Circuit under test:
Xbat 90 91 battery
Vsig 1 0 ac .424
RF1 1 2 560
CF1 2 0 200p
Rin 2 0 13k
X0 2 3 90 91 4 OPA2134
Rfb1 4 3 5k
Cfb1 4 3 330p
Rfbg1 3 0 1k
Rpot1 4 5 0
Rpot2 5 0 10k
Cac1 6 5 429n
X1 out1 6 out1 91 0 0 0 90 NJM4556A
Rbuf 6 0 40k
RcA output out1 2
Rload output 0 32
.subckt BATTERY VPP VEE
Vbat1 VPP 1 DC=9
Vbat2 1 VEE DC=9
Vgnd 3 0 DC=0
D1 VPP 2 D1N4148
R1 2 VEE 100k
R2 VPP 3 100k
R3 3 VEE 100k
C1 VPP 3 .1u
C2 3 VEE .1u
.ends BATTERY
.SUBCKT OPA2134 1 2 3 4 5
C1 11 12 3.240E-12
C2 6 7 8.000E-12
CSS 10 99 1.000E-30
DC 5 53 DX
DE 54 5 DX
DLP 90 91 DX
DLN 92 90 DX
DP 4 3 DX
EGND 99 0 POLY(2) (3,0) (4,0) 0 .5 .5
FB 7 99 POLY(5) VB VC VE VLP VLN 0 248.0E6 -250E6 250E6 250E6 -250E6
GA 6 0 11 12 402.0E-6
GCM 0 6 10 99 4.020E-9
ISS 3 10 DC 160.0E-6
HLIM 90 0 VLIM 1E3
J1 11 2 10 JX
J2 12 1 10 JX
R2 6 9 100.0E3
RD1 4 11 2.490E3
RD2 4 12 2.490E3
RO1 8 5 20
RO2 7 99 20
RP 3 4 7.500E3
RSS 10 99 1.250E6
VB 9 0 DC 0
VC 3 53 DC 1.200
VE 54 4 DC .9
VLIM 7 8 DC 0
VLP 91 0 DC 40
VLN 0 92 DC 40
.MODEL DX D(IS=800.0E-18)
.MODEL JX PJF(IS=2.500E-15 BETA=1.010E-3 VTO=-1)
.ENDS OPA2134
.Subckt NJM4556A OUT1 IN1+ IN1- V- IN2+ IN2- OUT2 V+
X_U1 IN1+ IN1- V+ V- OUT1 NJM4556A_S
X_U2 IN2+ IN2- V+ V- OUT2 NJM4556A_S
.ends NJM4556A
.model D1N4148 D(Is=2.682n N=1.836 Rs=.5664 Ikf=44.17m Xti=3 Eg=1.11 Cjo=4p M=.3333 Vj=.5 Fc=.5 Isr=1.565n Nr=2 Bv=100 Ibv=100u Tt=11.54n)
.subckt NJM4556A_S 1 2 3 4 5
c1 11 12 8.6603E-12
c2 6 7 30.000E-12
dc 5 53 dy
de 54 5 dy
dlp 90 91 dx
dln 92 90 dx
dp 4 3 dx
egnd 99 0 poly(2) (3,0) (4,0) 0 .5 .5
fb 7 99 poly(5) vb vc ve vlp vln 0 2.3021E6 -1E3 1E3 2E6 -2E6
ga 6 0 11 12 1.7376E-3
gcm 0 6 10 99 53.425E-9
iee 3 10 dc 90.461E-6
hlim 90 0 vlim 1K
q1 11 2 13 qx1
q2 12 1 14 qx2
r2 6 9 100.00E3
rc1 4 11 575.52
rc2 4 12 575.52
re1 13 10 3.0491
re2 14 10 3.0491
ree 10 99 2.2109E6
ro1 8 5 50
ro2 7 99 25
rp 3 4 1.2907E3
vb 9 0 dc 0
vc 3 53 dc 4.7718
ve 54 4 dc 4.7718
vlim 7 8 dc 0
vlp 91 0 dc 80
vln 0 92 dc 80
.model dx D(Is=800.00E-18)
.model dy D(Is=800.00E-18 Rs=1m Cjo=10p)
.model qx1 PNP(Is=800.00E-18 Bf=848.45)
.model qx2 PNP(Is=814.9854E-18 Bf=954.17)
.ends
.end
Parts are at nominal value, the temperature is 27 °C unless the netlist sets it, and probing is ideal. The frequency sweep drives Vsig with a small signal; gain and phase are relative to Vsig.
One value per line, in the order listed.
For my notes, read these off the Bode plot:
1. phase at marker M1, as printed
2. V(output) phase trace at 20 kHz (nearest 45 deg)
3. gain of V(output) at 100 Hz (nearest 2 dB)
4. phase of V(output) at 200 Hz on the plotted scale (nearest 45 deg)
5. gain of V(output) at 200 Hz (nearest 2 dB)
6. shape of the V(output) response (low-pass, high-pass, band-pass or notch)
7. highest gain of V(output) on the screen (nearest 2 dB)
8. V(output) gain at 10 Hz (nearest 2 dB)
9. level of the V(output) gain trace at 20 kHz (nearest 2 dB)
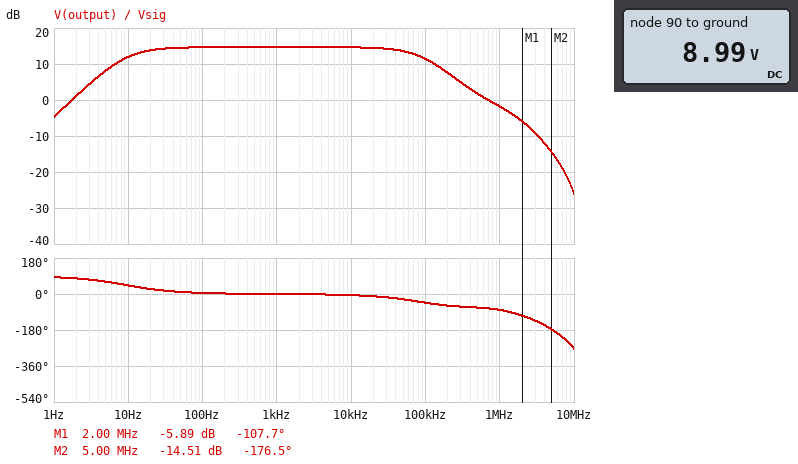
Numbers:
-107.7 deg
0 deg
14 dB
0 deg
14 dB
band-pass
14 dB
12 dB
14 dB
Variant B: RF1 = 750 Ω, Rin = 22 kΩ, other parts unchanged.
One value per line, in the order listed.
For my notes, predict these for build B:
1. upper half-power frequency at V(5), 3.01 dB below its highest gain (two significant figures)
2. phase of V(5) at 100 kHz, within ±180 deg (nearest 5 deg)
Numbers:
94 kHz
-45 deg
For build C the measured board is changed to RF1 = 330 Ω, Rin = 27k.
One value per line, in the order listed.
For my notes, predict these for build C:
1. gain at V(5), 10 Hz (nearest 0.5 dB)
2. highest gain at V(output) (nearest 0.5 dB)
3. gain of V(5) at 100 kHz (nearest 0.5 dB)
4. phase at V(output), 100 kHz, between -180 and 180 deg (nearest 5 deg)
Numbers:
15.5 dB
15.0 dB
12.0 dB
-40 deg
